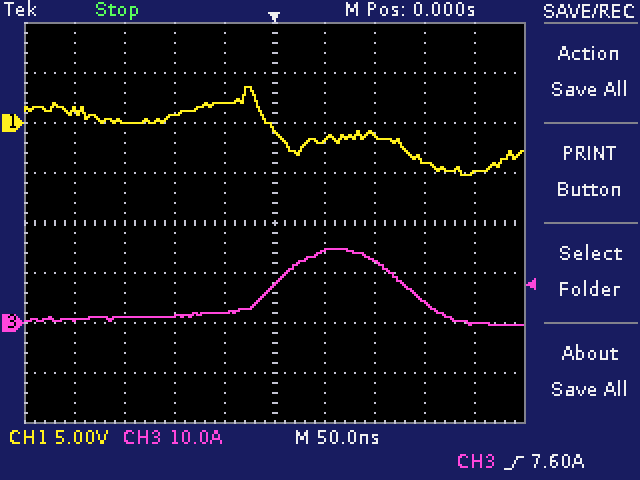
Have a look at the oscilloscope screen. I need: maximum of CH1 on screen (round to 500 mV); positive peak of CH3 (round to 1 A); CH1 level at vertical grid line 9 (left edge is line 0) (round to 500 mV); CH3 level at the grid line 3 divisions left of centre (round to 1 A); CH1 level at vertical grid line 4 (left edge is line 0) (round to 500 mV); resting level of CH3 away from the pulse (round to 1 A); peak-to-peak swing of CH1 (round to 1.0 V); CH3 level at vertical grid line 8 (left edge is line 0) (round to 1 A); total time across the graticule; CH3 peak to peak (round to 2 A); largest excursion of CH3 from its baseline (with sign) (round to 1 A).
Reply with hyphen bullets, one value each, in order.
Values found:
- 3.5 V
- 15 A
- -5.0 V
- 1 A
- 2.0 V
- 1 A
- 9.0 V
- 4 A
- 500 ns
- 16 A
- +14 A
